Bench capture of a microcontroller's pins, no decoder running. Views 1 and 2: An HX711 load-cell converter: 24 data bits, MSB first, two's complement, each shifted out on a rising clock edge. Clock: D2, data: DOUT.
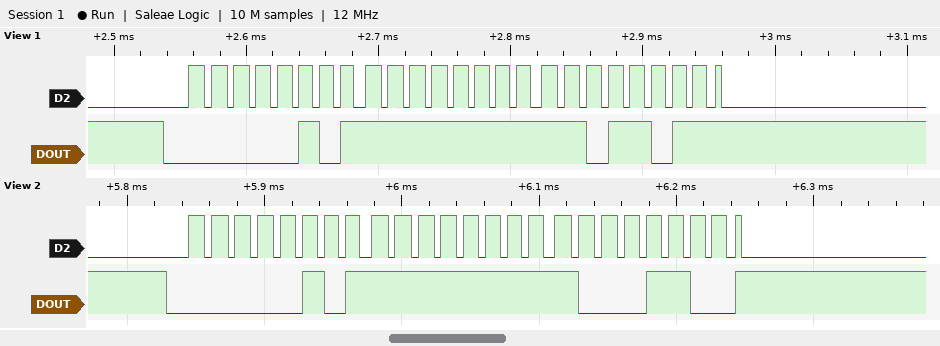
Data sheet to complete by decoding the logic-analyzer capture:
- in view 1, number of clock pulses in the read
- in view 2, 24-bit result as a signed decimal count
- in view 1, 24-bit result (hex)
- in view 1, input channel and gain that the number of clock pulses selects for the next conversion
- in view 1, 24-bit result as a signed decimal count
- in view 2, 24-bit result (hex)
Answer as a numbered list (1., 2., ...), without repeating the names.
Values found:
1. 25
2. 393100
3. 0x05FFDB
4. channel A, gain 128
5. 393179
6. 0x05FF8C
